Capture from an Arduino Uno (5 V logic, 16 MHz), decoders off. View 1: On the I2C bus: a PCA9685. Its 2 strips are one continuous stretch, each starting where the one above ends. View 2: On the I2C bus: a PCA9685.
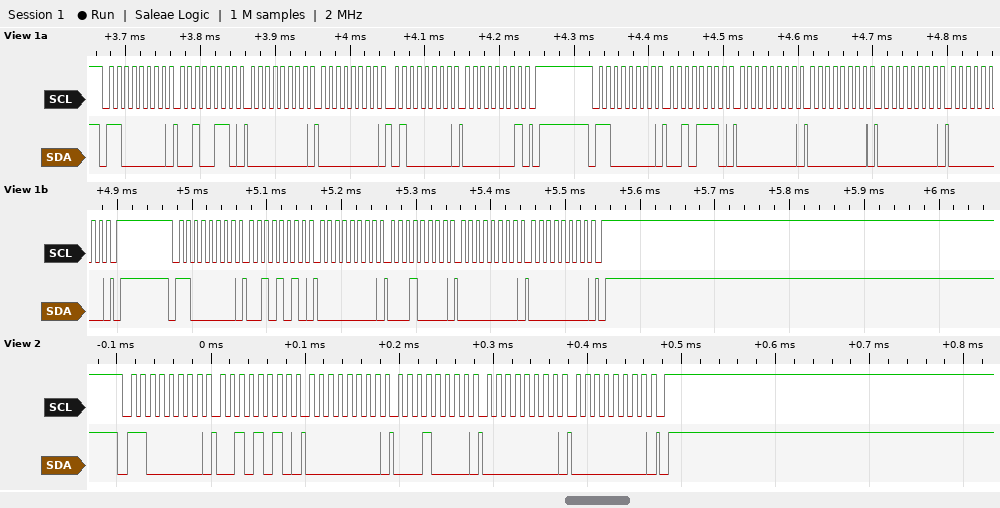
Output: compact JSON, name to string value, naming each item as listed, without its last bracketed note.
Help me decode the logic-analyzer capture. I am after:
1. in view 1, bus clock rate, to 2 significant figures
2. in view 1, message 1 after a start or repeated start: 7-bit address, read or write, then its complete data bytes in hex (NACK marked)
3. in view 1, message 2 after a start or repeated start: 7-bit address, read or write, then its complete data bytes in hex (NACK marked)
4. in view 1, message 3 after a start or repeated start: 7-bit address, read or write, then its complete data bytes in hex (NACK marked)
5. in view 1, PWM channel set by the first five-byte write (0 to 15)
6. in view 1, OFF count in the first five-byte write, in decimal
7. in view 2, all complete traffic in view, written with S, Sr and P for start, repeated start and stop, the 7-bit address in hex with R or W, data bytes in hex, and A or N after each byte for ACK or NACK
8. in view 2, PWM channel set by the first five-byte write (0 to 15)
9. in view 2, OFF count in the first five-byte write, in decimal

{"in view 1, bus clock rate, to 2 significant figures": "100 kHz", "in view 1, message 1 after a start or repeated start: 7-bit address, read or write, then its complete data bytes in hex": "0x60 write: 26 00 00 40 01", "in view 1, message 2 after a start or repeated start: 7-bit address, read or write, then its complete data bytes in hex": "0x60 write: 2E 00 00 00 00", "in view 1, message 3 after a start or repeated start: 7-bit address, read or write, then its complete data bytes in hex": "0x60 write: 2A 00 10 00 00", "in view 1, PWM channel set by the first five-byte write": "8", "in view 1, OFF count in the first five-byte write, in decimal": "320", "in view 2, all complete traffic in view, written with S, Sr and P for start, repeated start and stop, the 7-bit address in hex with R or W, data bytes in hex, and A or N after each byte for ACK or NACK": "S 60W A 2A A 00 A 10 A 00 A 00 A P", "in view 2, PWM channel set by the first five-byte write": "9", "in view 2, OFF count in the first five-byte write, in decimal": "0"}
